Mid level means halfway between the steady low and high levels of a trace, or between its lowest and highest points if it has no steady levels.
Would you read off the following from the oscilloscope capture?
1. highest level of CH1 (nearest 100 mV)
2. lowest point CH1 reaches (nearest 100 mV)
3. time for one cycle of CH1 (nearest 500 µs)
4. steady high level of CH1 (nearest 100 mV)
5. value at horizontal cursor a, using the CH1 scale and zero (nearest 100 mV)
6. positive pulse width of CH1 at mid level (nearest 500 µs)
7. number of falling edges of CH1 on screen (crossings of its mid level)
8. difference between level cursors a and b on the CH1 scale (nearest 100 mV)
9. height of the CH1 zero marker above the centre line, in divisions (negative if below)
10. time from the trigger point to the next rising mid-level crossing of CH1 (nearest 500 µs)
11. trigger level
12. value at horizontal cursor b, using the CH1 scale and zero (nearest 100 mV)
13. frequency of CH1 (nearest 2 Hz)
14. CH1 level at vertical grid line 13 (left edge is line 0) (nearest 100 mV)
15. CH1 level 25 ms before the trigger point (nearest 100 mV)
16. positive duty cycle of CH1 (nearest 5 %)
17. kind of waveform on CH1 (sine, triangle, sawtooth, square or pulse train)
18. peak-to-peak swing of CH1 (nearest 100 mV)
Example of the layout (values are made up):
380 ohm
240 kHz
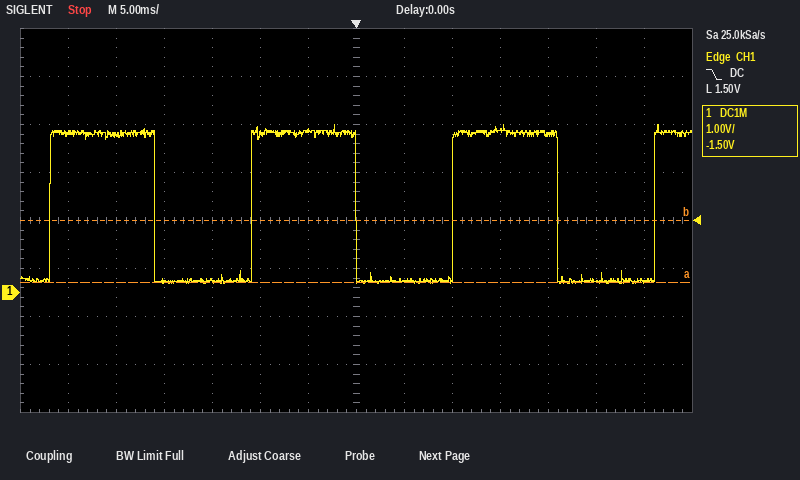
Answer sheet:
3.5 V
200 mV
21.0 ms
3.3 V
200 mV
11.0 ms
3
1.3 V
-1.5 div
10.0 ms
1.50 V
1.5 V
48 Hz
200 mV
3.3 V
50 %
square
3.3 V
